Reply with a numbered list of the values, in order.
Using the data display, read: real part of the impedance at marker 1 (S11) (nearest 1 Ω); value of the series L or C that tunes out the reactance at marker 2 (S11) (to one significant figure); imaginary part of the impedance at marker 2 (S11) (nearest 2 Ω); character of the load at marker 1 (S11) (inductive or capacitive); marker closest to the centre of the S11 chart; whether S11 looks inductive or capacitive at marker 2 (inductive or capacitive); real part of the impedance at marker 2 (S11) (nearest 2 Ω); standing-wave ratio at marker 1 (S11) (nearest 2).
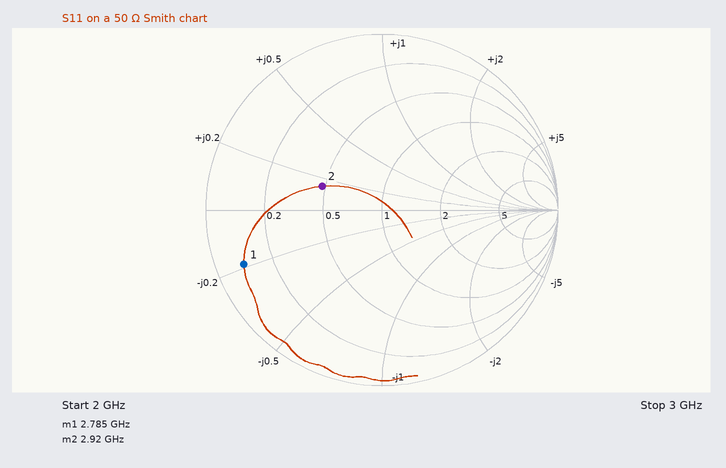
1. 4 Ω
2. 7 pF
3. +8 Ω
4. capacitive
5. marker 2
6. inductive
7. 24 Ω
8. 12
